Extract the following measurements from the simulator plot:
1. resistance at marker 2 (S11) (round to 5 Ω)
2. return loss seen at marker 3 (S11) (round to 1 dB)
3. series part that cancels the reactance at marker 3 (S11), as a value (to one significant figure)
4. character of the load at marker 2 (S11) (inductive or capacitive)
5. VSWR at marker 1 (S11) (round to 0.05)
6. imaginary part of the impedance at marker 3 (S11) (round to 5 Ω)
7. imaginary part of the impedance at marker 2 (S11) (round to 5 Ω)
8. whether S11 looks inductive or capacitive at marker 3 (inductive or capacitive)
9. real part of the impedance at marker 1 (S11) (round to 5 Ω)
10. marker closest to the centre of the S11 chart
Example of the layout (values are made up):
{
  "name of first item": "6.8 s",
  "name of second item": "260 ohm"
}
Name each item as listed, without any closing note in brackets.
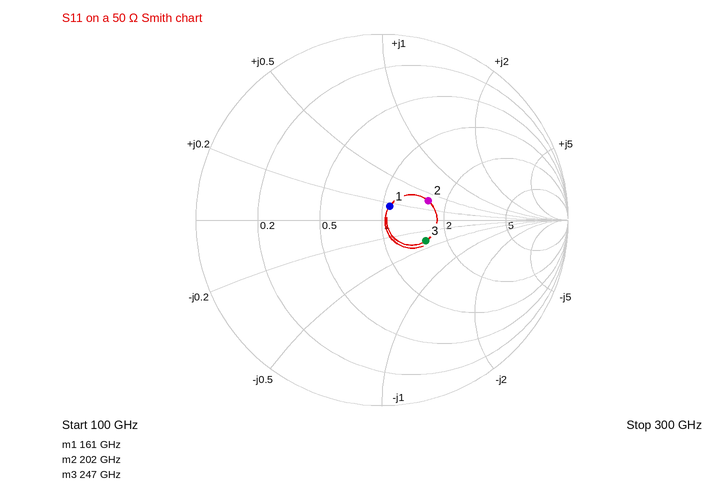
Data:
{
  "resistance at marker 2 (S11)": "80 Ω",
  "return loss seen at marker 3 (S11)": "12 dB",
  "series part that cancels the reactance at marker 3 (S11), as a value": "10 pH",
  "character of the load at marker 2 (S11)": "inductive",
  "VSWR at marker 1 (S11)": "1.20",
  "imaginary part of the impedance at marker 3 (S11)": "-20 Ω",
  "imaginary part of the impedance at marker 2 (S11)": "+20 Ω",
  "whether S11 looks inductive or capacitive at marker 3": "capacitive",
  "real part of the impedance at marker 1 (S11)": "55 Ω",
  "marker closest to the centre of the S11 chart": "marker 1"
}
